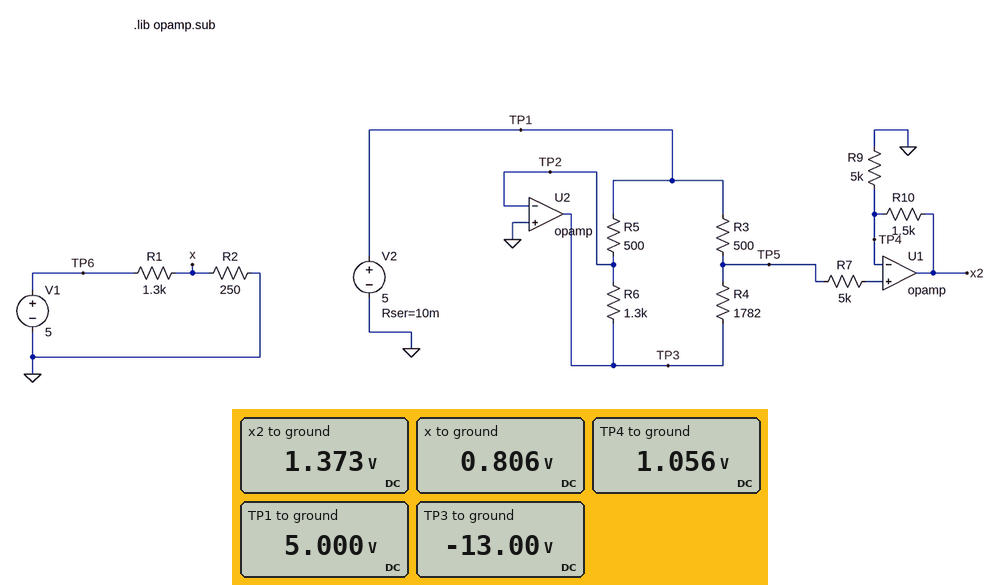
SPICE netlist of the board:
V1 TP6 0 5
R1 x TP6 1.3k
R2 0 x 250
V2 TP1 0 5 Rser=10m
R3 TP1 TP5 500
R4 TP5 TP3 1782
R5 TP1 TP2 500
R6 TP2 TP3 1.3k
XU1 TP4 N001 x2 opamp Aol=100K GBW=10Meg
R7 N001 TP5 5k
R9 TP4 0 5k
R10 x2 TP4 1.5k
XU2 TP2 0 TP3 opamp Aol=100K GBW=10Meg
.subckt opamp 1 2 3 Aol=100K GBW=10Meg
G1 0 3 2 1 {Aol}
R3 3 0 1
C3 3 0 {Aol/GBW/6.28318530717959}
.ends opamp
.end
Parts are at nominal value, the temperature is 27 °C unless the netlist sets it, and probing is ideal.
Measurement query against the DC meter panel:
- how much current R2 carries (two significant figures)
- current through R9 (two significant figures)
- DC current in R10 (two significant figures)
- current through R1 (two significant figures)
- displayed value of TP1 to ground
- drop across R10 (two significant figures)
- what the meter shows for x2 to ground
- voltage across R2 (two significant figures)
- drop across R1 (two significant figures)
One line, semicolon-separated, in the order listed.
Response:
3.2 mA; 210 µA; 210 µA; 3.2 mA; 5.000 V; 320 mV; 1.373 V; 810 mV; 4.2 V
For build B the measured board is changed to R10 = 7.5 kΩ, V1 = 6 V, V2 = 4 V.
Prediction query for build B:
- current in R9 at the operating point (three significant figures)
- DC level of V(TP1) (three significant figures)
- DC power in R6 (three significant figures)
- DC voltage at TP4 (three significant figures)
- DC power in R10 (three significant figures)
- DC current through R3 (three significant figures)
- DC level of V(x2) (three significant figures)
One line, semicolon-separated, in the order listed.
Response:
169 µA; 4.00 V; 83.2 mW; 845 mV; 214 µW; 6.31 mA; 2.11 V
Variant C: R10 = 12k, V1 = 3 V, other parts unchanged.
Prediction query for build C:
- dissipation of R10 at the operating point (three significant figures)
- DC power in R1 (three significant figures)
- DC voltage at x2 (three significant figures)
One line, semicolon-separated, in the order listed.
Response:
535 µW; 4.87 mW; 3.59 V
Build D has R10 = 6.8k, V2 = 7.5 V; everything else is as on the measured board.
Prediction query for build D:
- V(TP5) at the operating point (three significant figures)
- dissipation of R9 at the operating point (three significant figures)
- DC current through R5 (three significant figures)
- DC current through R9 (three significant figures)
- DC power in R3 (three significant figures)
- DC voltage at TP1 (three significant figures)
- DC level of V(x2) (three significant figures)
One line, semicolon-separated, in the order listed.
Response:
1.58 V; 502 µW; 15.0 mA; 317 µA; 70.0 mW; 7.50 V; 3.74 V
